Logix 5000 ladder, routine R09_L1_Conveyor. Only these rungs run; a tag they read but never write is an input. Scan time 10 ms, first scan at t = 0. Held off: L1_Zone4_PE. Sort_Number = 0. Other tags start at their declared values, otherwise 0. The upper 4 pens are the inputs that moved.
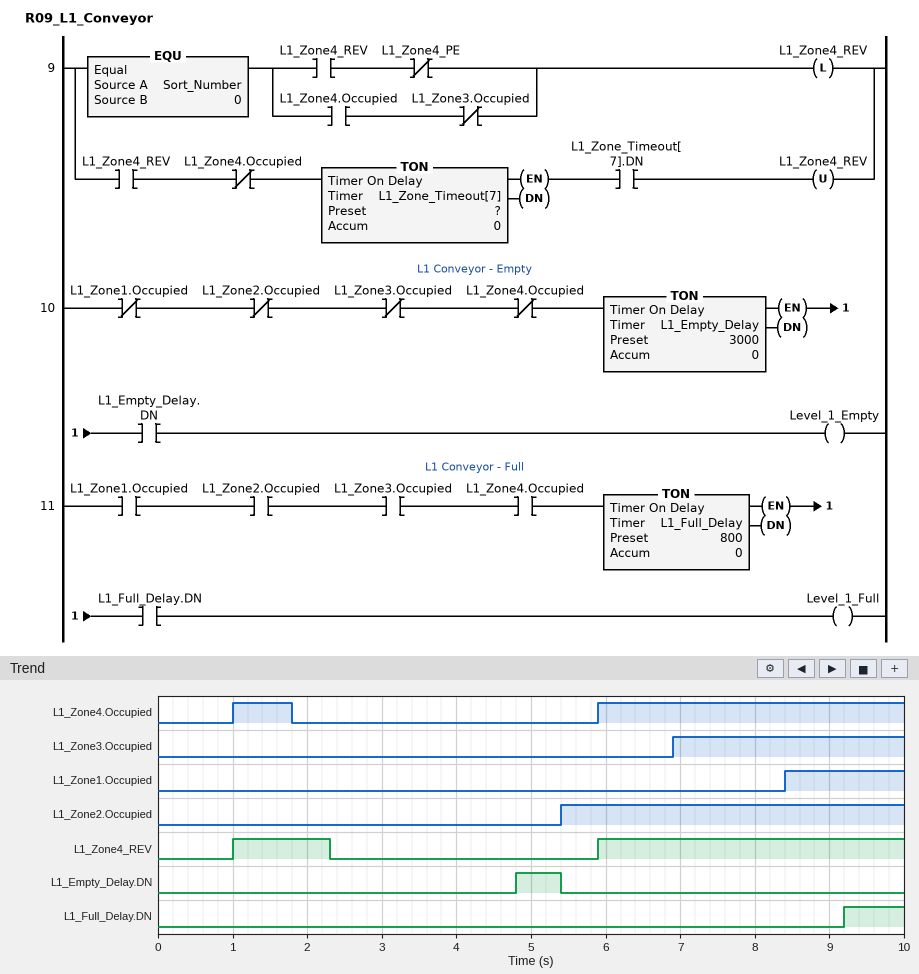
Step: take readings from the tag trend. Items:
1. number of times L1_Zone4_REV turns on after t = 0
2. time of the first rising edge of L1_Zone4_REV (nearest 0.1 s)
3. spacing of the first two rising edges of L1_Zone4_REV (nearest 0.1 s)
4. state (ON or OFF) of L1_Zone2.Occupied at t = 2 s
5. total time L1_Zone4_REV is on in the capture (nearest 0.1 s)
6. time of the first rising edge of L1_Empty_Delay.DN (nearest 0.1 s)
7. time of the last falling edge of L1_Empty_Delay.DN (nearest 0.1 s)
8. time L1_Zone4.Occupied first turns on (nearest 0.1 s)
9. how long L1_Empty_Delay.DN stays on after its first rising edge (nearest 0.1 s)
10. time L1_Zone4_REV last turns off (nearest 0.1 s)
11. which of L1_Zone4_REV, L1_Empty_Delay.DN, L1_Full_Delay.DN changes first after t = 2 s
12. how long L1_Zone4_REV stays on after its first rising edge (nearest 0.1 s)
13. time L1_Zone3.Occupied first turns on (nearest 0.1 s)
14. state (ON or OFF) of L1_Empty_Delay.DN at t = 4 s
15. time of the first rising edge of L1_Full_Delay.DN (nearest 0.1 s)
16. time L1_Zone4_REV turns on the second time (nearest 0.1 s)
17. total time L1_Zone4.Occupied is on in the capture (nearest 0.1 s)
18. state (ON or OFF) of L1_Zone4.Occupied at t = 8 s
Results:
2
1.0 s
4.9 s
OFF
5.4 s
4.8 s
5.4 s
1.0 s
0.6 s
2.3 s
L1_Zone4_REV
1.3 s
6.9 s
OFF
9.2 s
5.9 s
4.9 s
ON
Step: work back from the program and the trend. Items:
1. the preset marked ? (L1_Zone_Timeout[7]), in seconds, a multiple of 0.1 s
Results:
0.5 s
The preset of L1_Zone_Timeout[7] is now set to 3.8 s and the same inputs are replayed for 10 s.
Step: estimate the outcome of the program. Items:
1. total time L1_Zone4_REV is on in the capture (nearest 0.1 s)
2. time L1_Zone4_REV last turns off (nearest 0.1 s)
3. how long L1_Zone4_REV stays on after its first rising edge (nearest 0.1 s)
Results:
8.7 s
5.6 s
4.6 s
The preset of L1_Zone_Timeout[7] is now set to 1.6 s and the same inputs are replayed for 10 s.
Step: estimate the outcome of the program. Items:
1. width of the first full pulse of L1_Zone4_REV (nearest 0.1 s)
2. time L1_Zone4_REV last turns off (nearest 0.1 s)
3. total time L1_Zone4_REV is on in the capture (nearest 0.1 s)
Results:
2.4 s
3.4 s
6.5 s
